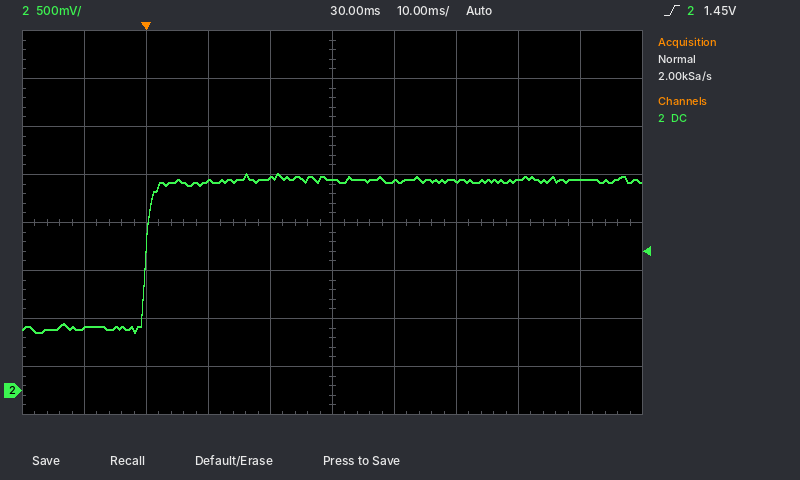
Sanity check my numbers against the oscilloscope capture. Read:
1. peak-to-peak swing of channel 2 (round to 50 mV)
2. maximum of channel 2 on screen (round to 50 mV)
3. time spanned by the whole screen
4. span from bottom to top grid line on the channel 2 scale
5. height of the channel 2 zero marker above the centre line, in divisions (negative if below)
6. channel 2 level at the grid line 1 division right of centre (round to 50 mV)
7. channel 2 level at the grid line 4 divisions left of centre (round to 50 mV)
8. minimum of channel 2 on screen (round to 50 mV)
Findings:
1.65 V
2.25 V
100 ms
4 V
-3.5 div
2.20 V
650 mV
600 mV
